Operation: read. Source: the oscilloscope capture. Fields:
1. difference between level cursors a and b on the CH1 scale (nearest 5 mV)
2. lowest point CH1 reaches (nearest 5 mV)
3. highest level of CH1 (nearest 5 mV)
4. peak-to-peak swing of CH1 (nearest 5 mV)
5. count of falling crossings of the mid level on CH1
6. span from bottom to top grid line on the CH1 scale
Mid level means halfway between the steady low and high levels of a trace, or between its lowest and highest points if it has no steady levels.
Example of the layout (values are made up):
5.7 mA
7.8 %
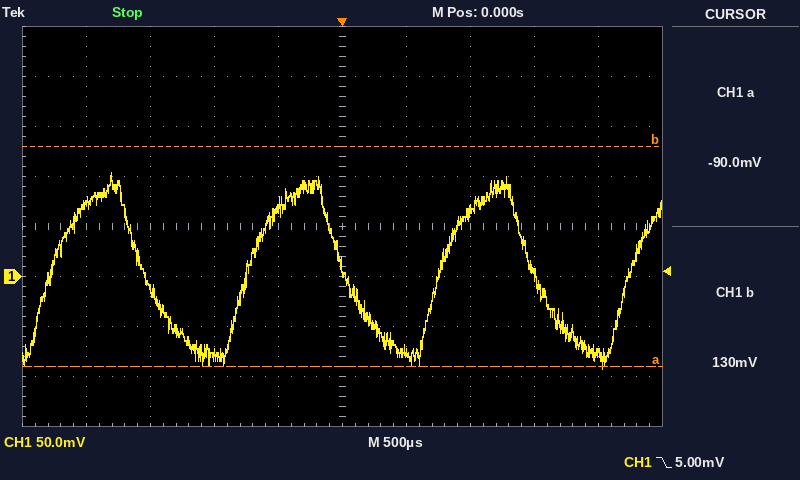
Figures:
220 mV
-90 mV
105 mV
195 mV
3
400 mV
